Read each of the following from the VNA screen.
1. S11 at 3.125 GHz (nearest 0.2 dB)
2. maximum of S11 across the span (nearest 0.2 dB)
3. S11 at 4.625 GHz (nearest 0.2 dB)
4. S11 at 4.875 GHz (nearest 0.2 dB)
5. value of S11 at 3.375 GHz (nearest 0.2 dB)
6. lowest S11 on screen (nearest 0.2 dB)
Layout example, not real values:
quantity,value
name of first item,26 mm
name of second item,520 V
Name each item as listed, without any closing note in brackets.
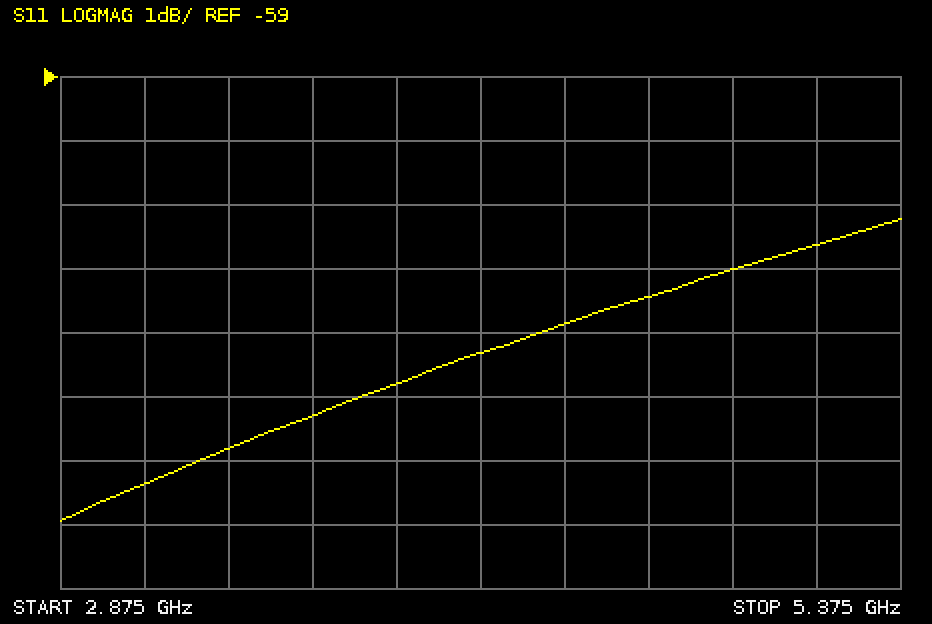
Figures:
quantity,value
S11 at 3.125 GHz,-65.4 dB
maximum of S11 across the span,-61.2 dB
S11 at 4.625 GHz,-62.4 dB
S11 at 4.875 GHz,-62.0 dB
value of S11 at 3.375 GHz,-64.8 dB
lowest S11 on screen,-66.0 dB
